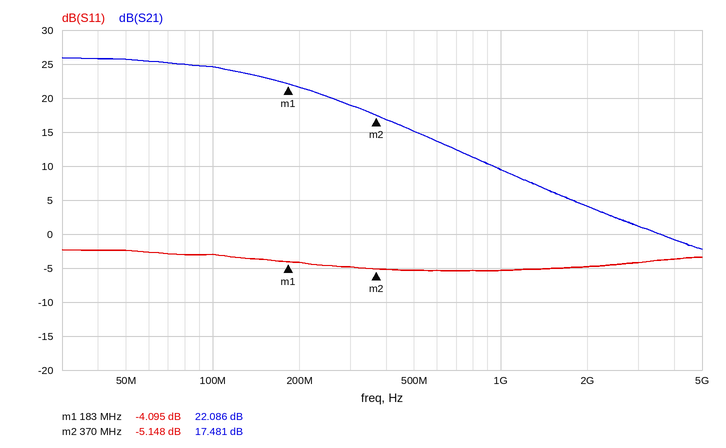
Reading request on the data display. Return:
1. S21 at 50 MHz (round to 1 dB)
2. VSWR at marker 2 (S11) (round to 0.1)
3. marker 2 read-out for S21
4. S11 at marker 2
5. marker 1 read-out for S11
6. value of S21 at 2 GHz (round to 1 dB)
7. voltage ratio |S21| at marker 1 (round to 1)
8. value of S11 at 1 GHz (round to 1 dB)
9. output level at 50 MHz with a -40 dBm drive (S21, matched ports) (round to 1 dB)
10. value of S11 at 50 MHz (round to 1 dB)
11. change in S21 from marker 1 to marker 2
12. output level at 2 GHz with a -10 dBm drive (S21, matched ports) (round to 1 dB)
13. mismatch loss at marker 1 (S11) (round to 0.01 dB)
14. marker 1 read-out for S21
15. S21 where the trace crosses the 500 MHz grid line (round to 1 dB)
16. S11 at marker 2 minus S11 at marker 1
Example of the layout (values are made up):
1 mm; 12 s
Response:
26 dB; 3.5; 17.481 dB; -5.148 dB; -4.095 dB; 4 dB; 13; -5 dB; -14 dBm; -2 dB; -4.605 dB; -6 dBm; 2.14 dB; 22.086 dB; 15 dB; -1.053 dB
